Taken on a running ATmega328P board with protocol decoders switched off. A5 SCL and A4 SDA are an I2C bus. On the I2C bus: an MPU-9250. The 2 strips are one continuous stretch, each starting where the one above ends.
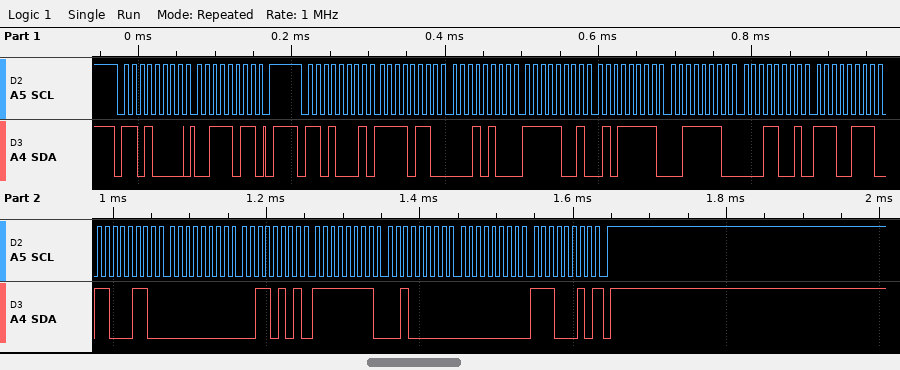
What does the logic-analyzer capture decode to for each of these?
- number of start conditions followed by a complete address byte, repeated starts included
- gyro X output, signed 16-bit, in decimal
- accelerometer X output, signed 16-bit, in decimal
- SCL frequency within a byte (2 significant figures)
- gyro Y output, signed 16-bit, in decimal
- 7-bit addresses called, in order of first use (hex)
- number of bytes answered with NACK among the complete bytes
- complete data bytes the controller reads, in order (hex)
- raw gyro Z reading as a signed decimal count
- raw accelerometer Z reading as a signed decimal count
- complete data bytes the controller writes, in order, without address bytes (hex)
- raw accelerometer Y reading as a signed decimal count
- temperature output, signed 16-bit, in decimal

2
53
-2540
100 kHz
-224
0x68
1
F6 14 F9 5F 3E 19 E7 C6 00 35 FF 20 00 E2
226
15897
3B
-1697
-6202
